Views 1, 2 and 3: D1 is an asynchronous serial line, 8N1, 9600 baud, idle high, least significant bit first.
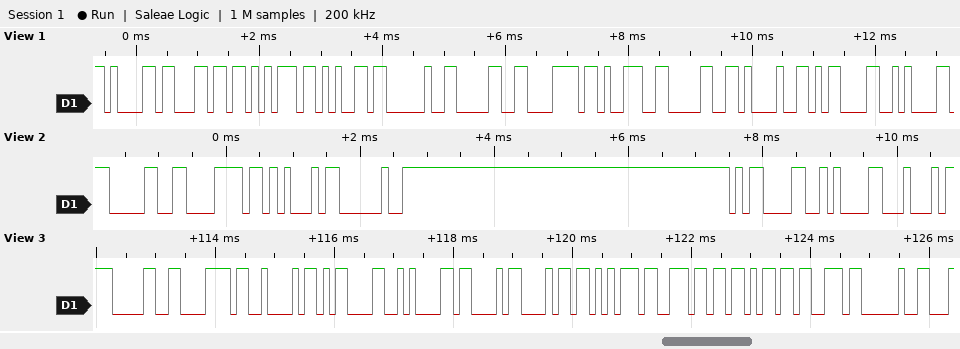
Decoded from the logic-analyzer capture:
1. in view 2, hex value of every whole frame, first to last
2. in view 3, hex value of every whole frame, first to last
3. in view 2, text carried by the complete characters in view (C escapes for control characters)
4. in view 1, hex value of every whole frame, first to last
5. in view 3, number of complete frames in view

30 78 45 20 0D 0A 44
30 78 42 0D 0A 43 68 75 6E 6B 73 20
"0xE \r\nD"
61 6C 75 65 20 30 78 39 30 21 0D 0A
12
